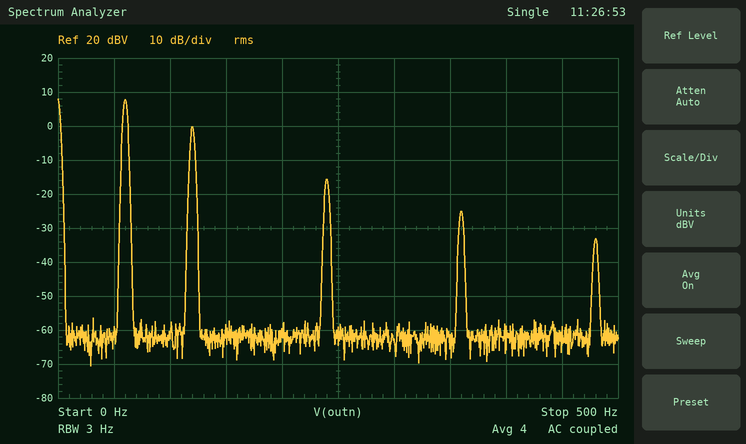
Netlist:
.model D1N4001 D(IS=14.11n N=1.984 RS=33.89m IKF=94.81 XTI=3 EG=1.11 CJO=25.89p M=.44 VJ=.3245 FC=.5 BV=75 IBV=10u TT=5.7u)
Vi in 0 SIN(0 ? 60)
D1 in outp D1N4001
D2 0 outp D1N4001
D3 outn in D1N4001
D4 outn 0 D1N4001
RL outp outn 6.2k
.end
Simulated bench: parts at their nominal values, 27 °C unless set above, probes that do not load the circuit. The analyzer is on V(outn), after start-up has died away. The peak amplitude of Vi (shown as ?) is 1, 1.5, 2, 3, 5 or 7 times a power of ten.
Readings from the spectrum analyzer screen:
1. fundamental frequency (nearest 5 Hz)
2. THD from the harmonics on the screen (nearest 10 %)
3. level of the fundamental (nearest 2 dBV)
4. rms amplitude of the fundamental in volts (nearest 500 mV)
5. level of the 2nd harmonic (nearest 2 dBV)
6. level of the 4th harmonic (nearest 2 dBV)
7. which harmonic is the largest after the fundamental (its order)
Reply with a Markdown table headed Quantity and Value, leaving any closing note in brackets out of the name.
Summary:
| Quantity | Value |
|---|---|
| fundamental frequency | 60 Hz |
| THD from the harmonics on the screen | 40 % |
| level of the fundamental | 8 dBV |
| rms amplitude of the fundamental in volts | 2.5 V |
| level of the 2nd harmonic | 0 dBV |
| level of the 4th harmonic | -16 dBV |
| which harmonic is the largest after the fundamental | 2 |
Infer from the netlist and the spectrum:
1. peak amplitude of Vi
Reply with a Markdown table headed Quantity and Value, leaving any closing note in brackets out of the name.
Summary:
| Quantity | Value |
|---|---|
| peak amplitude of Vi | 7 V |
